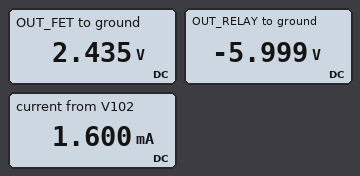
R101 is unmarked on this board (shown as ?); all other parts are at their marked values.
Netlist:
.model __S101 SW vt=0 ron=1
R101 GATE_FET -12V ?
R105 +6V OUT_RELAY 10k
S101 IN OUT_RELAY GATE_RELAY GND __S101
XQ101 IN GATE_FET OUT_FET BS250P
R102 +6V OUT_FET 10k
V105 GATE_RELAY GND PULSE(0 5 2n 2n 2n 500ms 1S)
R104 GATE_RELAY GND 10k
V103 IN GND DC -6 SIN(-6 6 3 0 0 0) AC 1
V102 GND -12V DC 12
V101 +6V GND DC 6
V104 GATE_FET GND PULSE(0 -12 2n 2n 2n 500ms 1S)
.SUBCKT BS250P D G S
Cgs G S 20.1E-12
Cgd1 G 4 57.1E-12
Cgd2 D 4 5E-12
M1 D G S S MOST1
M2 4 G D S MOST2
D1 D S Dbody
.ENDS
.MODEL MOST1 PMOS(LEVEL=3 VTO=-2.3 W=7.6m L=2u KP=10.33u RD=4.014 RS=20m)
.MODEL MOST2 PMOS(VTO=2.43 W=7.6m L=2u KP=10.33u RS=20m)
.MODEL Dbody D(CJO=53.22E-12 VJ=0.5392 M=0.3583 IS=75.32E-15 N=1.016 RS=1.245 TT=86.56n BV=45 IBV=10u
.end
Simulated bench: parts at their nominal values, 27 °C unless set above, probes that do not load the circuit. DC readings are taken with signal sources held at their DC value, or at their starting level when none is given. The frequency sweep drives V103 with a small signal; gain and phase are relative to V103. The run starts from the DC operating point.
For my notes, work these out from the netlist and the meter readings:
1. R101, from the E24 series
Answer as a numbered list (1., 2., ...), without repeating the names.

1. 7.5 kΩ
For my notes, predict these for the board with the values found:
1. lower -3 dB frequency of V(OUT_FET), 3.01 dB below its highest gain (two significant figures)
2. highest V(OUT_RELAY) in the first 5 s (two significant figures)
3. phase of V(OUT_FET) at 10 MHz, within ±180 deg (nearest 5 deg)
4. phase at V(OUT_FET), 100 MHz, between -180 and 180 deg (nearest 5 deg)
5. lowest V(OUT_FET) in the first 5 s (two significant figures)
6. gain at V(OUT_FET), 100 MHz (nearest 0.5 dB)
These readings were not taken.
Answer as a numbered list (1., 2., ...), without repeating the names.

1. 20 MHz
2. 6.0 V
3. 65 deg
4. 10 deg
5. -9.4 V
6. -7.0 dB
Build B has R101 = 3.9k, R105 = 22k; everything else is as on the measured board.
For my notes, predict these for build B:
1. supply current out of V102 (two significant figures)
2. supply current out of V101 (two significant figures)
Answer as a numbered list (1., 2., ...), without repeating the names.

1. 3.1 mA
2. 900 µA
